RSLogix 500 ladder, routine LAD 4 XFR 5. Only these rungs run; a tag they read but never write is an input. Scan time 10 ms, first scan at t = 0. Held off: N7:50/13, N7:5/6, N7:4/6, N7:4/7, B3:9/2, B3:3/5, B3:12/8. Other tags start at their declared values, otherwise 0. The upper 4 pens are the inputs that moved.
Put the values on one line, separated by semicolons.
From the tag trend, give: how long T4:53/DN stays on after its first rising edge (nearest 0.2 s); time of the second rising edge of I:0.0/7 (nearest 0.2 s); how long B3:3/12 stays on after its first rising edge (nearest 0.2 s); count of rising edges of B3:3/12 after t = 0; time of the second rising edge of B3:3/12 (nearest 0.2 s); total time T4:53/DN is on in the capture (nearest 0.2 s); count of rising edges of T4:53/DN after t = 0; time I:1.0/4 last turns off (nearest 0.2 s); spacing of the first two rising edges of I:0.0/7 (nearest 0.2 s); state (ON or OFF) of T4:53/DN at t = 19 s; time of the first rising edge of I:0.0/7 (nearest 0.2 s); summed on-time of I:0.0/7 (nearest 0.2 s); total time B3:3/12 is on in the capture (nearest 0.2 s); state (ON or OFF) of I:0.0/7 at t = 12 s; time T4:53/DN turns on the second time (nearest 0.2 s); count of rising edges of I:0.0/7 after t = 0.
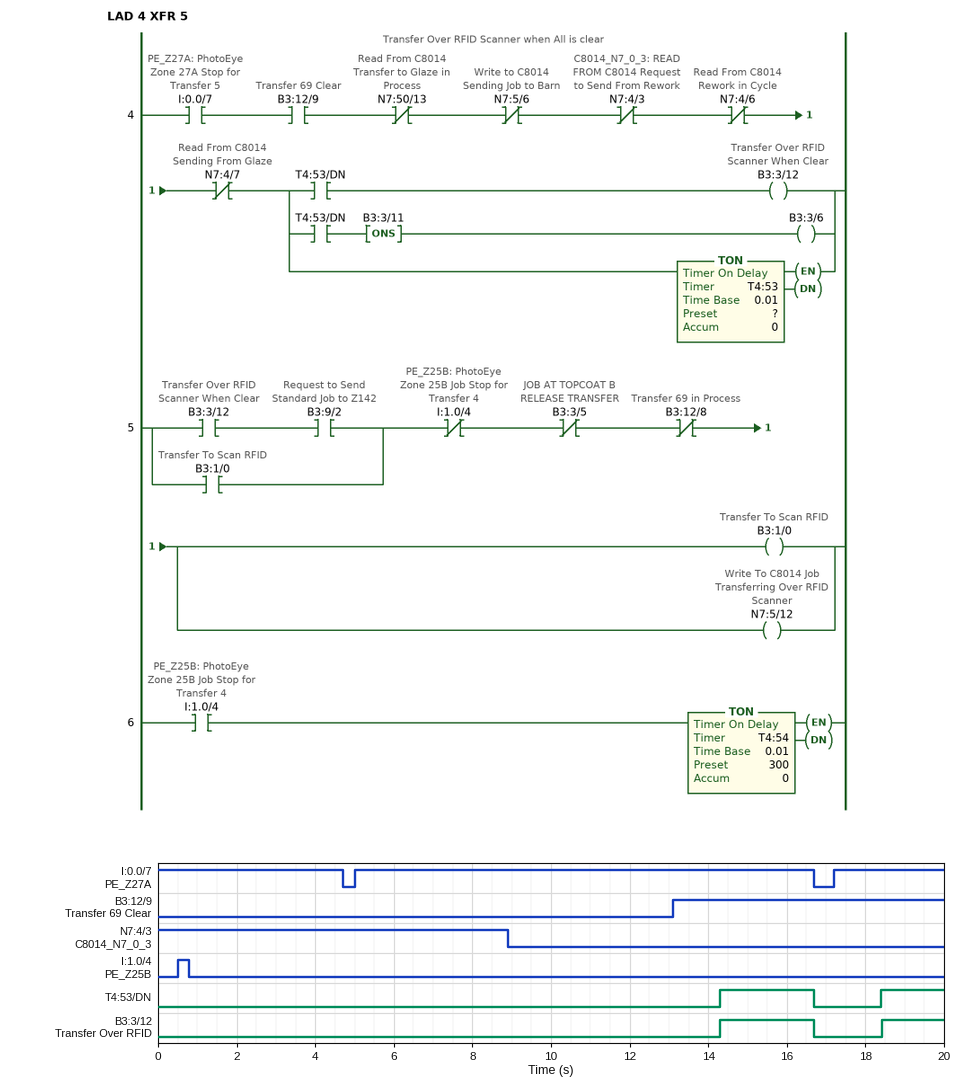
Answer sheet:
2.4 s; 17.2 s; 2.4 s; 2; 18.4 s; 4.0 s; 2; 0.8 s; 12.2 s; ON; 5.0 s; 19.2 s; 4.0 s; ON; 18.4 s; 2
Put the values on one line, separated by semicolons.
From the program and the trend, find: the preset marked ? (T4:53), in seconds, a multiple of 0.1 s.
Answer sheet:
1.2 s
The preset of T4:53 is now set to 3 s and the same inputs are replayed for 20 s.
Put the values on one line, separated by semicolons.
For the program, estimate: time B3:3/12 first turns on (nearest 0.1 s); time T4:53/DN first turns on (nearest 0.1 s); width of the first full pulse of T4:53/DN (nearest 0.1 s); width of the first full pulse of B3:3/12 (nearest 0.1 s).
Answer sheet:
16.1 s; 16.1 s; 0.6 s; 0.6 s
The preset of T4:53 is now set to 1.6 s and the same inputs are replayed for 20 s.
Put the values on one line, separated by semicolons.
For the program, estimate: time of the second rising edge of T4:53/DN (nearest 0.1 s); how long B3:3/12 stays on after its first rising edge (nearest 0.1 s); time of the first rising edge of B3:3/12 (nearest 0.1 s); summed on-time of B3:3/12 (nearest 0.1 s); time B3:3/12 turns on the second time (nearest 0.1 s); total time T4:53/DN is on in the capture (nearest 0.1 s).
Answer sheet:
18.8 s; 2.0 s; 14.7 s; 3.2 s; 18.8 s; 3.2 s
